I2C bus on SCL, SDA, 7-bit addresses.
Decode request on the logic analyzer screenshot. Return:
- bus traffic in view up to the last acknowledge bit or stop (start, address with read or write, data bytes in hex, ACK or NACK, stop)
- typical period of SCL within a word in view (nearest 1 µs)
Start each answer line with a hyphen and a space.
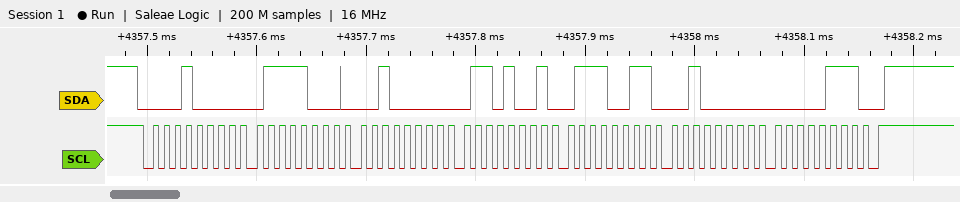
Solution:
- start, address 08 write ACK, 78 ACK, 20 ACK, 69 ACK, 73 ACK, 20 ACK, 07 ACK, stop
- 10 µs
